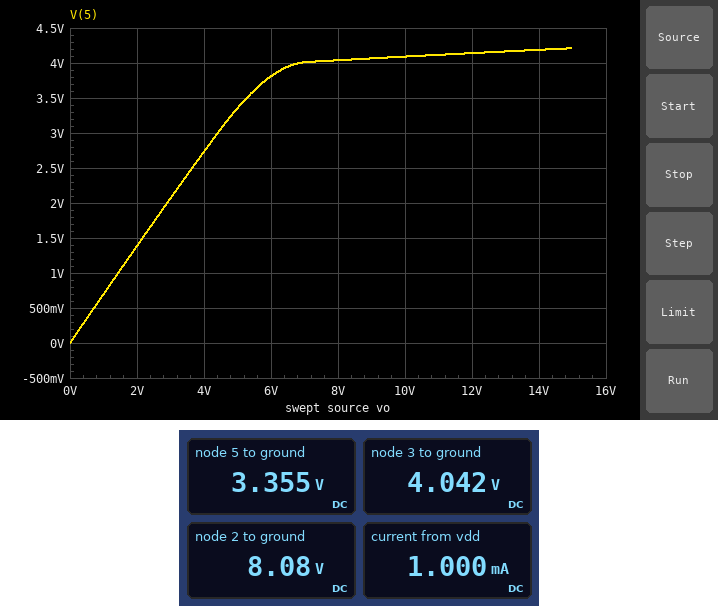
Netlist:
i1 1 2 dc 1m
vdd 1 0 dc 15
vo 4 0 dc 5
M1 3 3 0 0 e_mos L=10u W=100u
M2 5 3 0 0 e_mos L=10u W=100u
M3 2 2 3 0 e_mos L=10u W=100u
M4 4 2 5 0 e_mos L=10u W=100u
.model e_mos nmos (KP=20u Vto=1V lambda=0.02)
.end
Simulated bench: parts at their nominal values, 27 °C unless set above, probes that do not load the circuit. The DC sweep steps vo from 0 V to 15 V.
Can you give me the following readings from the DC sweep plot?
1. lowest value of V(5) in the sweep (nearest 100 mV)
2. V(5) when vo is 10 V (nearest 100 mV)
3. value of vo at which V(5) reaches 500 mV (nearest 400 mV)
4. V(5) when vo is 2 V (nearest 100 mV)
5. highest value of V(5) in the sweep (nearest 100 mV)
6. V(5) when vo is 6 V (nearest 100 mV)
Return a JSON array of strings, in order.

["0 V", "4.1 V", "800 mV", "1.4 V", "4.2 V", "3.8 V"]
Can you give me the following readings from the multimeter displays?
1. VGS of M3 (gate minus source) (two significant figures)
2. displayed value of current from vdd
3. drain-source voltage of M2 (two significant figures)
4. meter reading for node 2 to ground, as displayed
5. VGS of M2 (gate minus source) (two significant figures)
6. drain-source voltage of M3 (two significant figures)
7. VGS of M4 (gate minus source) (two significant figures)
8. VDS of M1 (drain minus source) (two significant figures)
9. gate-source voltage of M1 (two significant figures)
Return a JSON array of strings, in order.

["4.0 V", "1.000 mA", "3.4 V", "8.08 V", "4.0 V", "4.0 V", "4.7 V", "4.0 V", "4.0 V"]
